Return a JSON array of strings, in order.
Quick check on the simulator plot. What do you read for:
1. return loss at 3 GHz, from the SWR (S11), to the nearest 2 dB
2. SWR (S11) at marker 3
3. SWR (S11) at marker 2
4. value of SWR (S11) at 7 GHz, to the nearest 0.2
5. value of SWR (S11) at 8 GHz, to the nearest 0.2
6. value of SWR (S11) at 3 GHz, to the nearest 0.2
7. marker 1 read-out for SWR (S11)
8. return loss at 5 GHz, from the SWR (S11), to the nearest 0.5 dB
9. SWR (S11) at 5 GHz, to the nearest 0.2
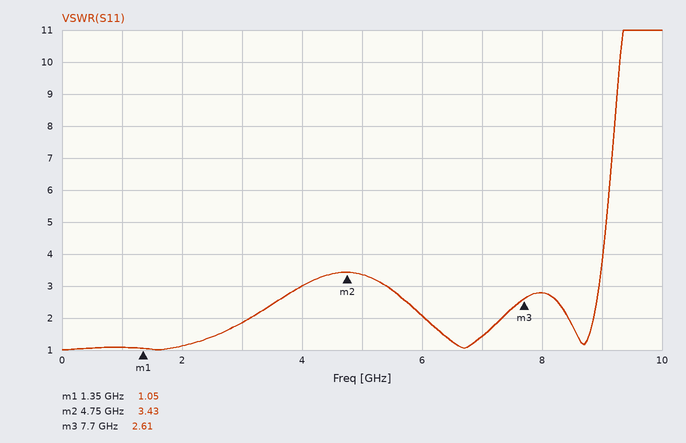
["10 dB", "2.61", "3.43", "1.4", "2.8", "1.8", "1.05", "5.5 dB", "3.4"]
